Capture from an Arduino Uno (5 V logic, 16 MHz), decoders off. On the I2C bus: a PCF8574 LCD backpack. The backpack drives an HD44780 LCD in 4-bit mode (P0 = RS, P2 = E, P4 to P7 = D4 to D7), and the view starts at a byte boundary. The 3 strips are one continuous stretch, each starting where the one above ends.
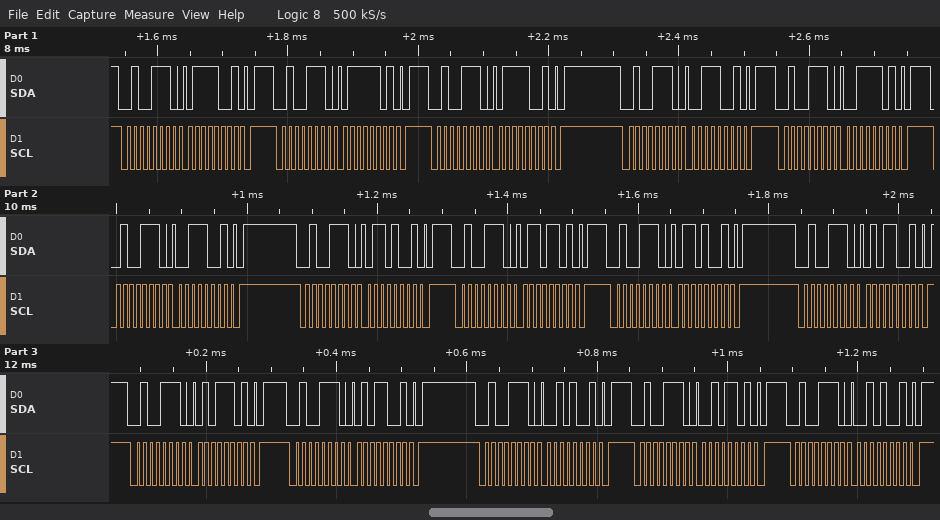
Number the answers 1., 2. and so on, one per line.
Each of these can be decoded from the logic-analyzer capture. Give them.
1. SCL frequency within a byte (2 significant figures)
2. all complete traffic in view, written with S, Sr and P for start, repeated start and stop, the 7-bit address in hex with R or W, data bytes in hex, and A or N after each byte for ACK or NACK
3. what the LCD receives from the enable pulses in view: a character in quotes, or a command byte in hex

1. 100 kHz
2. S 27W A 79 A P S 27W A 7D A P S 27W A 79 A P S 27W A 39 A P S 27W A 3D A P S 27W A 39 A P S 27W A 69 A P S 27W A 6D A P S 27W A 69 A P S 27W A 59 A P S 27W A 5D A P S 27W A 59 A P S 27W A 29 A P S 27W A 2D A P S 27W A 29 A P
3. 's' 'e'
